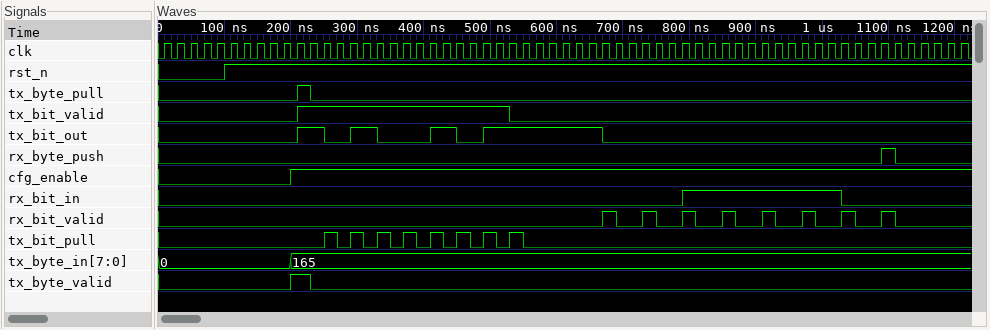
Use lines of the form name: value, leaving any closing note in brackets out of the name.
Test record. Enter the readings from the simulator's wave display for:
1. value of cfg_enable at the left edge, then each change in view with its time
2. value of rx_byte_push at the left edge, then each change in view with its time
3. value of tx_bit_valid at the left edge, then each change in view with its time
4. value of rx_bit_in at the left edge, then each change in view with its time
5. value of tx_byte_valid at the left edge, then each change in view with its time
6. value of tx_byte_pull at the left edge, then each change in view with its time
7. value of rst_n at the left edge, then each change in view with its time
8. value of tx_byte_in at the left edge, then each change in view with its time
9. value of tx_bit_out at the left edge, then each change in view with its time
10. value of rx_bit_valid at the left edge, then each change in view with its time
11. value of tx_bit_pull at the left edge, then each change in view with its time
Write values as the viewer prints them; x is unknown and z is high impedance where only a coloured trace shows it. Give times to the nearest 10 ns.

value of cfg_enable at the left edge, then each change in view with its time: 0, 1 at 200 ns
value of rx_byte_push at the left edge, then each change in view with its time: 0, 1 at 1090 ns, 0 at 1110 ns
value of tx_bit_valid at the left edge, then each change in view with its time: 0, 1 at 210 ns, 0 at 530 ns
value of rx_bit_in at the left edge, then each change in view with its time: 0, 1 at 790 ns, 0 at 1030 ns
value of tx_byte_valid at the left edge, then each change in view with its time: 0, 1 at 200 ns, 0 at 230 ns
value of tx_byte_pull at the left edge, then each change in view with its time: 0, 1 at 210 ns, 0 at 230 ns
value of rst_n at the left edge, then each change in view with its time: 0, 1 at 100 ns
value of tx_byte_in at the left edge, then each change in view with its time: 0, 165 at 200 ns
value of tx_bit_out at the left edge, then each change in view with its time: 0, 1 at 210 ns, 0 at 250 ns, 1 at 290 ns, 0 at 330 ns, 1 at 410 ns, 0 at 450 ns, 1 at 490 ns, 0 at 670 ns
value of rx_bit_valid at the left edge, then each change in view with its time: 0, 1 at 670 ns, 0 at 690 ns, 1 at 730 ns, 0 at 750 ns, 1 at 790 ns, 0 at 810 ns, 1 at 850 ns, 0 at 870 ns, 1 at 910 ns, 0 at 930 ns, 1 at 970 ns, 0 at 990 ns, 1 at 1030 ns, 0 at 1050 ns, 1 at 1090 ns, 0 at 1110 ns
value of tx_bit_pull at the left edge, then each change in view with its time: 0, 1 at 250 ns, 0 at 270 ns, 1 at 290 ns, 0 at 310 ns, 1 at 330 ns, 0 at 350 ns, 1 at 370 ns, 0 at 390 ns, 1 at 410 ns, 0 at 430 ns, 1 at 450 ns, 0 at 470 ns, 1 at 490 ns, 0 at 510 ns, 1 at 530 ns, 0 at 550 ns
